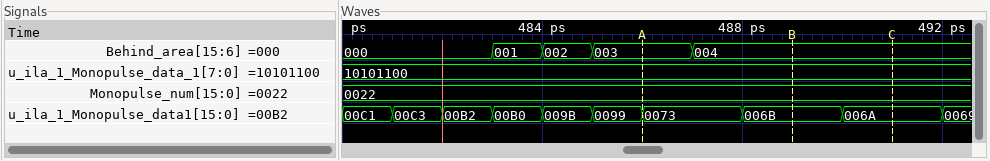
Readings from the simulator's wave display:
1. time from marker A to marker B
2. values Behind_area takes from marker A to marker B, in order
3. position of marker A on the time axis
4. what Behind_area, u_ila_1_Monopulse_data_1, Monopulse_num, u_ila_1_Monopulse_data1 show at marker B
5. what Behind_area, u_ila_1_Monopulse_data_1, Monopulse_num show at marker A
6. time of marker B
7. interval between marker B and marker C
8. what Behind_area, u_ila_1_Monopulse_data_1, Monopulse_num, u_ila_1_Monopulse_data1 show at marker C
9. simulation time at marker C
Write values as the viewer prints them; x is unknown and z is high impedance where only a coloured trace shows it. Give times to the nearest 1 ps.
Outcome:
3 ps
003, 004
486 ps
Behind_area=004, u_ila_1_Monopulse_data_1=10101100, Monopulse_num=0022, u_ila_1_Monopulse_data1=006B
Behind_area=003, u_ila_1_Monopulse_data_1=10101100, Monopulse_num=0022
489 ps
2 ps
Behind_area=004, u_ila_1_Monopulse_data_1=10101100, Monopulse_num=0022, u_ila_1_Monopulse_data1=006A
491 ps
